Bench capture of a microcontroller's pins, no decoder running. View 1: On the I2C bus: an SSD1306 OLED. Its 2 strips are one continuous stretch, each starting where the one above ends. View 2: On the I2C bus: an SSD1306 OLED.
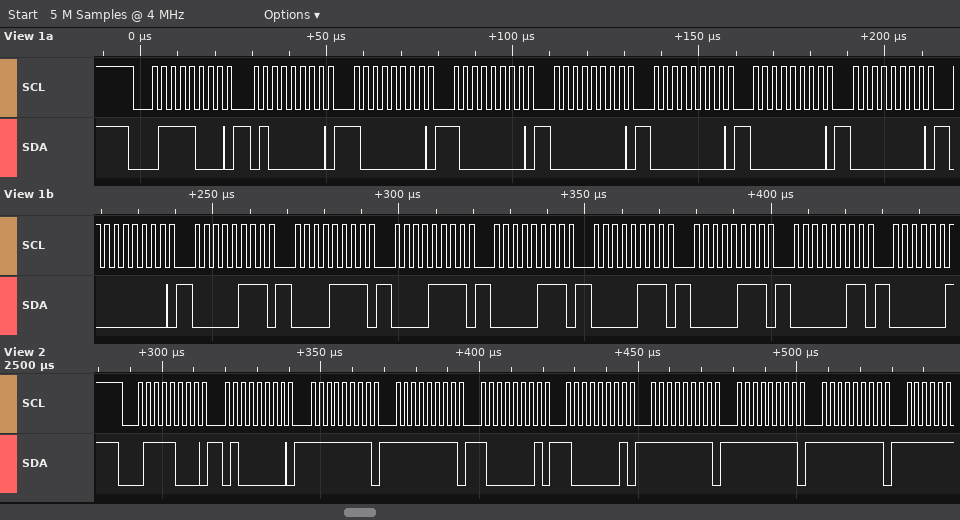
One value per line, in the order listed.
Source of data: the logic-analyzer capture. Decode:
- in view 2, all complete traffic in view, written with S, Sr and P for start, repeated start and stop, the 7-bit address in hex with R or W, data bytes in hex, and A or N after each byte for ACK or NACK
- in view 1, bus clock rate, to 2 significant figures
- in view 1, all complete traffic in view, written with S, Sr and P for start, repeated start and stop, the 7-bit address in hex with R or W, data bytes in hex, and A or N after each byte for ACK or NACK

S 3CW A 40 A FF A FF A 81 A 81 A FF A FF A FF A
400 kHz
S 3CW A 40 A 80 A 80 A 00 A 00 A 00 A 00 A 00 A 07 A 0F A 0F A 07 A 07 A 07 A 03 A
